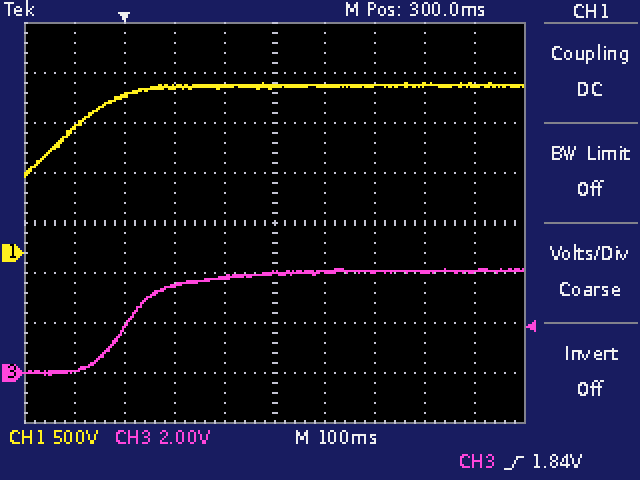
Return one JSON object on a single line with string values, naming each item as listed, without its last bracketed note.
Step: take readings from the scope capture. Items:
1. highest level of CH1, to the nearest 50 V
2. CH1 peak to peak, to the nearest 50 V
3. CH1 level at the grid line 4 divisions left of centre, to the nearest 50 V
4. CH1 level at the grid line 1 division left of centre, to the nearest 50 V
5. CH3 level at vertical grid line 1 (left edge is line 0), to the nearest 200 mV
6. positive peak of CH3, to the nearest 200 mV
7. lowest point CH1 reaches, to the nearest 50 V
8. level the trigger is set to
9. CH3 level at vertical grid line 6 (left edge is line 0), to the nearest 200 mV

{"highest level of CH1, to the nearest 50 V": "1.70 kV", "CH1 peak to peak, to the nearest 50 V": "950 V", "CH1 level at the grid line 4 divisions left of centre, to the nearest 50 V": "1.25 kV", "CH1 level at the grid line 1 division left of centre, to the nearest 50 V": "1.65 kV", "CH3 level at vertical grid line 1 (left edge is line 0), to the nearest 200 mV": "0.0 V", "positive peak of CH3, to the nearest 200 mV": "4.2 V", "lowest point CH1 reaches, to the nearest 50 V": "750 V", "level the trigger is set to": "1.84 V", "CH3 level at vertical grid line 6 (left edge is line 0), to the nearest 200 mV": "4.0 V"}
